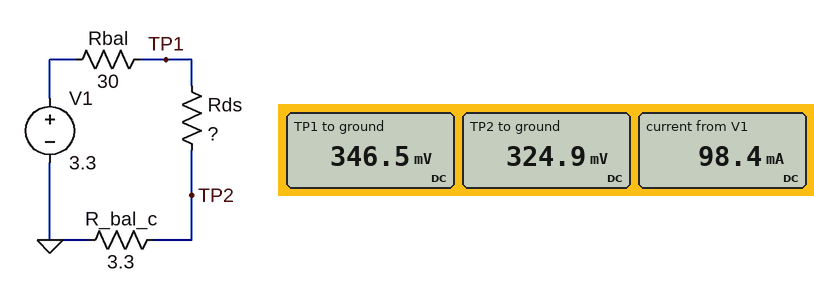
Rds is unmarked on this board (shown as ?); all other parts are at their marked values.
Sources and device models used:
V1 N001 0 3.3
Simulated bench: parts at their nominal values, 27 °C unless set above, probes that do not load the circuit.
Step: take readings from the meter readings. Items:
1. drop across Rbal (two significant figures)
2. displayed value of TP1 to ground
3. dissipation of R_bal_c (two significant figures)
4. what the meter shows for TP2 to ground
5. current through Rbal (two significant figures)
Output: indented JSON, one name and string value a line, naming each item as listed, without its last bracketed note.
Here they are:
{
  "drop across Rbal": "3.0 V",
  "displayed value of TP1 to ground": "346.5 mV",
  "dissipation of R_bal_c": "32 mW",
  "what the meter shows for TP2 to ground": "324.9 mV",
  "current through Rbal": "98 mA"
}
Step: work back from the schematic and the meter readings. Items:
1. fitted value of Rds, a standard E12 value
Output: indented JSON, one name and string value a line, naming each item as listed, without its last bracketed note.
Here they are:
{
  "fitted value of Rds, a standard E12 value": "0.22 Ω"
}
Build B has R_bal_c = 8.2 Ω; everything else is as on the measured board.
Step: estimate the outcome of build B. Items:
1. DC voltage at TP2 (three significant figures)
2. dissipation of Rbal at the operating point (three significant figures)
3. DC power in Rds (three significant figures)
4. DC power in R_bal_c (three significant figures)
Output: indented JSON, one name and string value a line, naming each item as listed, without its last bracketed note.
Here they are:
{
  "DC voltage at TP2": "704 mV",
  "dissipation of Rbal at the operating point": "221 mW",
  "DC power in Rds": "1.62 mW",
  "DC power in R_bal_c": "60.5 mW"
}
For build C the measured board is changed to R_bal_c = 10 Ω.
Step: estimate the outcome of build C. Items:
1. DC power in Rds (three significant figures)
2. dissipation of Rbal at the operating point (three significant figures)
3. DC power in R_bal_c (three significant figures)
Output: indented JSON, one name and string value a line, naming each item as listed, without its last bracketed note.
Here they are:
{
  "DC power in Rds": "1.48 mW",
  "dissipation of Rbal at the operating point": "202 mW",
  "DC power in R_bal_c": "67.3 mW"
}
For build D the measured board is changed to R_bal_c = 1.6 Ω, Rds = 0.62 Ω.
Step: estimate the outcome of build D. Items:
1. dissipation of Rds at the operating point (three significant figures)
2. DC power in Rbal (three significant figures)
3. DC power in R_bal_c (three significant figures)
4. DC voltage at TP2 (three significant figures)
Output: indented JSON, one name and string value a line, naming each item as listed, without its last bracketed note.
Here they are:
{
  "dissipation of Rds at the operating point": "6.50 mW",
  "DC power in Rbal": "315 mW",
  "DC power in R_bal_c": "16.8 mW",
  "DC voltage at TP2": "164 mV"
}
